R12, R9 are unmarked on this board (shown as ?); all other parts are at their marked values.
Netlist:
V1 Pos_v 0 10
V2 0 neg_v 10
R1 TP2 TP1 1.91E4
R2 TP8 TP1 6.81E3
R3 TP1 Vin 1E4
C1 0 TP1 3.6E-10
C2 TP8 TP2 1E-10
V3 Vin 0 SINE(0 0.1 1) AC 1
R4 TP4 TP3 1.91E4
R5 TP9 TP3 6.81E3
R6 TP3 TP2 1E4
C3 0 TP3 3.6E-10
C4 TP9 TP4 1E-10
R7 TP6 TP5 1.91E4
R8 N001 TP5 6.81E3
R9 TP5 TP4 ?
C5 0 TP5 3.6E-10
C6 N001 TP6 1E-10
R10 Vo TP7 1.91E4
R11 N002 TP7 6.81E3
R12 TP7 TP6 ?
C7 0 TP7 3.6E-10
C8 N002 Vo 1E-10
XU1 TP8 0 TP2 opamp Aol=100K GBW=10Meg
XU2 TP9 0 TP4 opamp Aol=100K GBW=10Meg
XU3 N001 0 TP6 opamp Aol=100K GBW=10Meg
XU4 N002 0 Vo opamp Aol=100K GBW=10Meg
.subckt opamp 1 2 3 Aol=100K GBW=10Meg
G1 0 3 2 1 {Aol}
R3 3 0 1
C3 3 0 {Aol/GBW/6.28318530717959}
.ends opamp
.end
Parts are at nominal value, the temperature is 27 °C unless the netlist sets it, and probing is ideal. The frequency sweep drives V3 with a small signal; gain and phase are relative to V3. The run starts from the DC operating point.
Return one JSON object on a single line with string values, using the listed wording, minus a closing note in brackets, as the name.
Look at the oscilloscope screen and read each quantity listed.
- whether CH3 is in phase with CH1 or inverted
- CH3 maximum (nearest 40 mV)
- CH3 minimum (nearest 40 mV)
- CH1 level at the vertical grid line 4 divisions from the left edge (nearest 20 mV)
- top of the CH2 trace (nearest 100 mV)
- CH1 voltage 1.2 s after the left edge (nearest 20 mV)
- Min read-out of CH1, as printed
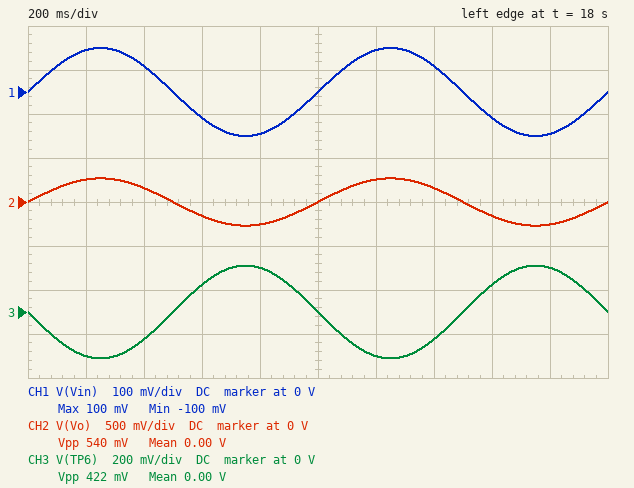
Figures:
{"whether CH3 is in phase with CH1 or inverted": "inverted", "CH3 maximum": "200 mV", "CH3 minimum": "-200 mV", "CH1 level at the vertical grid line 4 divisions from the left edge": "-100 mV", "top of the CH2 trace": "300 mV", "CH1 voltage 1.2 s after the left edge": "100 mV", "Min read-out of CH1, as printed": "-100 mV"}
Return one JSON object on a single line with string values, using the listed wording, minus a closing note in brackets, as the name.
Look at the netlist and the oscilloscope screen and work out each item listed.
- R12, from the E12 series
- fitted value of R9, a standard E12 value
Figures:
{"R12, from the E12 series": "15 kΩ", "fitted value of R9, a standard E12 value": "33 kΩ"}
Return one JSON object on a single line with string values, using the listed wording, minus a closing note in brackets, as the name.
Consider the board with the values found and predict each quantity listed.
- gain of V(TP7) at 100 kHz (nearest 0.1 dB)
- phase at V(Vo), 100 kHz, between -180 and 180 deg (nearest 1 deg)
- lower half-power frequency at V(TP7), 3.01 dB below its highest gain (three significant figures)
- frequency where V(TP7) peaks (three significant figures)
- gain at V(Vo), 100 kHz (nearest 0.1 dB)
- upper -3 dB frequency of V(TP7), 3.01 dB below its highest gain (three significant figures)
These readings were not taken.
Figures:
{"gain of V(TP7) at 100 kHz": "-29.2 dB", "phase at V(Vo), 100 kHz, between -180 and 180 deg": "-90 deg", "lower half-power frequency at V(TP7), 3.01 dB below its highest gain": "18.8 kHz", "frequency where V(TP7) peaks": "37.5 kHz", "gain at V(Vo), 100 kHz": "-22.0 dB", "upper -3 dB frequency of V(TP7), 3.01 dB below its highest gain": "59.1 kHz"}
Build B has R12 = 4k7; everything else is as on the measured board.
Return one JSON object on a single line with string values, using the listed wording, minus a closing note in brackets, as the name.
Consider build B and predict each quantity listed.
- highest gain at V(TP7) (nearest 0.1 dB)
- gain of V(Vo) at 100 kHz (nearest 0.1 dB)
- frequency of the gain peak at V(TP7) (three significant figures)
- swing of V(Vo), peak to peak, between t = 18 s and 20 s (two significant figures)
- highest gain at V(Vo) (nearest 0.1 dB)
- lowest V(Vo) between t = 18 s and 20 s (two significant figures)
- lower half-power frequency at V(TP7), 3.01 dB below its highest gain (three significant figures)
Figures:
{"highest gain at V(TP7)": "-3.2 dB", "gain of V(Vo) at 100 kHz": "-15.4 dB", "frequency of the gain peak at V(TP7)": "31.8 kHz", "swing of V(Vo), peak to peak, between t = 18 s and 20 s": "1.7 V", "highest gain at V(Vo)": "18.7 dB", "lowest V(Vo) between t = 18 s and 20 s": "-860 mV", "lower half-power frequency at V(TP7), 3.01 dB below its highest gain": "14.8 kHz"}
